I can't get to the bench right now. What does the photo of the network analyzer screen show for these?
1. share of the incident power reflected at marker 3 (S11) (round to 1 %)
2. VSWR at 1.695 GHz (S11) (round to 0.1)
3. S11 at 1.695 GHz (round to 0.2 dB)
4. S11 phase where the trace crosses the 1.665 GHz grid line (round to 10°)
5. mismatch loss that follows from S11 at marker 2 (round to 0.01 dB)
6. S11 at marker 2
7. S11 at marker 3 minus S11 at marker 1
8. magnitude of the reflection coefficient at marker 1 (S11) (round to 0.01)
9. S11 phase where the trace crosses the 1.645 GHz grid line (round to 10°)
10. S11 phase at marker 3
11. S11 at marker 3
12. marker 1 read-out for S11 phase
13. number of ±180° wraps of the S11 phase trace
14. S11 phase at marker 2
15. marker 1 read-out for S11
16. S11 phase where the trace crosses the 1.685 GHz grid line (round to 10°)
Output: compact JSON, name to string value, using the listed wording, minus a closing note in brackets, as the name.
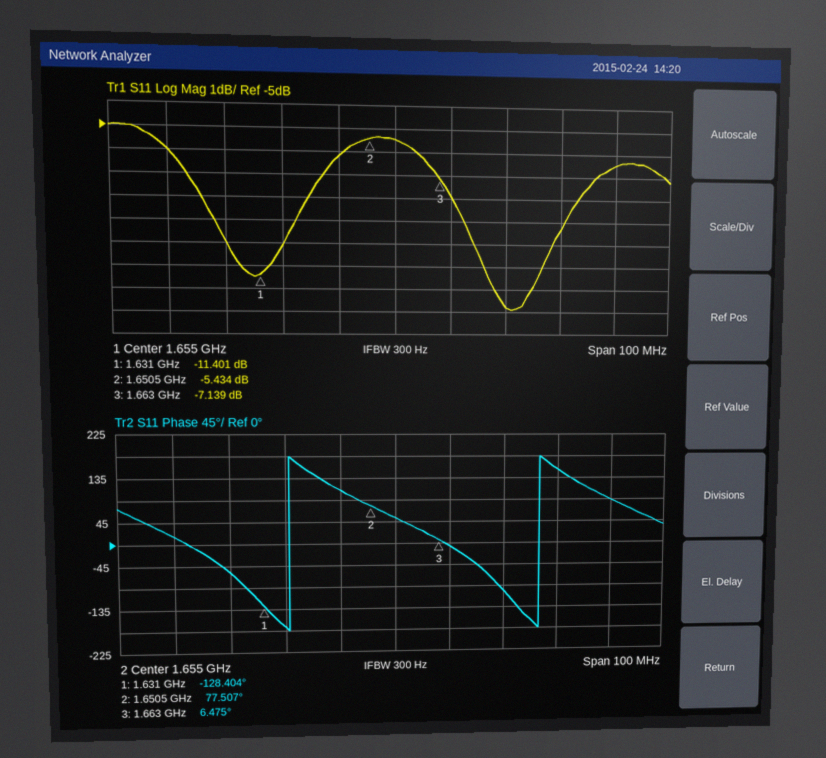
{"share of the incident power reflected at marker 3 (S11)": "19 %", "VSWR at 1.695 GHz (S11)": "2.8", "S11 at 1.695 GHz": "-6.4 dB", "S11 phase where the trace crosses the 1.665 GHz grid line": "-10°", "mismatch loss that follows from S11 at marker 2": "1.46 dB", "S11 at marker 2": "-5.434 dB", "S11 at marker 3 minus S11 at marker 1": "4.262 dB", "magnitude of the reflection coefficient at marker 1 (S11)": "0.27", "S11 phase where the trace crosses the 1.645 GHz grid line": "110°", "S11 phase at marker 3": "6.475°", "S11 at marker 3": "-7.139 dB", "marker 1 read-out for S11 phase": "-128.404°", "number of ±180° wraps of the S11 phase trace": "2", "S11 phase at marker 2": "77.507°", "marker 1 read-out for S11": "-11.401 dB", "S11 phase where the trace crosses the 1.685 GHz grid line": "150°"}
